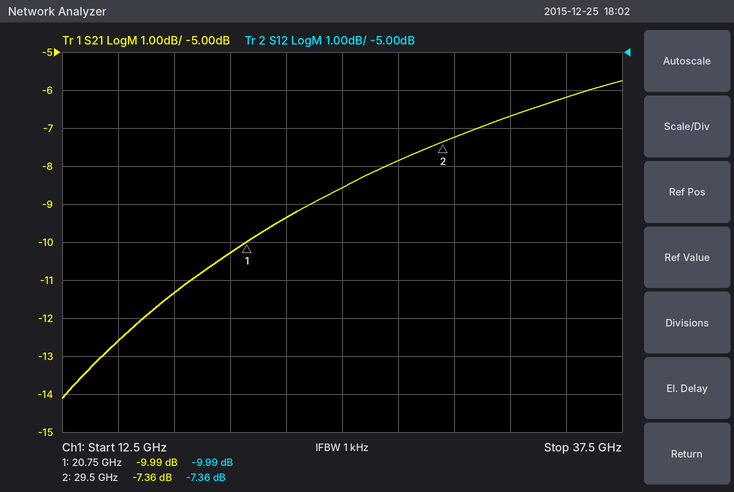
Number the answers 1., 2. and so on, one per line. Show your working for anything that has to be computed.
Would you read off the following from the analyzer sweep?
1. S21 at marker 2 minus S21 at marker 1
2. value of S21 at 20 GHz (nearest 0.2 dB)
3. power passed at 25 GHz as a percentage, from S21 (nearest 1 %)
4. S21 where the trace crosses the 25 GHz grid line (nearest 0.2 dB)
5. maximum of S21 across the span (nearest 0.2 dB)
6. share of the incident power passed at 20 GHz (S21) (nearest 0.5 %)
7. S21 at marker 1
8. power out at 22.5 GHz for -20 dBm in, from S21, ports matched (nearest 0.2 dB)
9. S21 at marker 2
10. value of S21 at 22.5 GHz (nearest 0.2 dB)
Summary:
1. -7.36 − (-9.99) = 2.63 dB
2. -10.2 dB
3. 10^(-8.6/10) ≈ 14 %
4. -8.6 dB
5. -5.8 dB
6. 10^(-10.2/10) ≈ 9.5 %
7. -9.99 dB
8. -20 dBm + (-9.4 dB) = -29.4 dBm
9. -7.36 dB
10. -9.4 dB
